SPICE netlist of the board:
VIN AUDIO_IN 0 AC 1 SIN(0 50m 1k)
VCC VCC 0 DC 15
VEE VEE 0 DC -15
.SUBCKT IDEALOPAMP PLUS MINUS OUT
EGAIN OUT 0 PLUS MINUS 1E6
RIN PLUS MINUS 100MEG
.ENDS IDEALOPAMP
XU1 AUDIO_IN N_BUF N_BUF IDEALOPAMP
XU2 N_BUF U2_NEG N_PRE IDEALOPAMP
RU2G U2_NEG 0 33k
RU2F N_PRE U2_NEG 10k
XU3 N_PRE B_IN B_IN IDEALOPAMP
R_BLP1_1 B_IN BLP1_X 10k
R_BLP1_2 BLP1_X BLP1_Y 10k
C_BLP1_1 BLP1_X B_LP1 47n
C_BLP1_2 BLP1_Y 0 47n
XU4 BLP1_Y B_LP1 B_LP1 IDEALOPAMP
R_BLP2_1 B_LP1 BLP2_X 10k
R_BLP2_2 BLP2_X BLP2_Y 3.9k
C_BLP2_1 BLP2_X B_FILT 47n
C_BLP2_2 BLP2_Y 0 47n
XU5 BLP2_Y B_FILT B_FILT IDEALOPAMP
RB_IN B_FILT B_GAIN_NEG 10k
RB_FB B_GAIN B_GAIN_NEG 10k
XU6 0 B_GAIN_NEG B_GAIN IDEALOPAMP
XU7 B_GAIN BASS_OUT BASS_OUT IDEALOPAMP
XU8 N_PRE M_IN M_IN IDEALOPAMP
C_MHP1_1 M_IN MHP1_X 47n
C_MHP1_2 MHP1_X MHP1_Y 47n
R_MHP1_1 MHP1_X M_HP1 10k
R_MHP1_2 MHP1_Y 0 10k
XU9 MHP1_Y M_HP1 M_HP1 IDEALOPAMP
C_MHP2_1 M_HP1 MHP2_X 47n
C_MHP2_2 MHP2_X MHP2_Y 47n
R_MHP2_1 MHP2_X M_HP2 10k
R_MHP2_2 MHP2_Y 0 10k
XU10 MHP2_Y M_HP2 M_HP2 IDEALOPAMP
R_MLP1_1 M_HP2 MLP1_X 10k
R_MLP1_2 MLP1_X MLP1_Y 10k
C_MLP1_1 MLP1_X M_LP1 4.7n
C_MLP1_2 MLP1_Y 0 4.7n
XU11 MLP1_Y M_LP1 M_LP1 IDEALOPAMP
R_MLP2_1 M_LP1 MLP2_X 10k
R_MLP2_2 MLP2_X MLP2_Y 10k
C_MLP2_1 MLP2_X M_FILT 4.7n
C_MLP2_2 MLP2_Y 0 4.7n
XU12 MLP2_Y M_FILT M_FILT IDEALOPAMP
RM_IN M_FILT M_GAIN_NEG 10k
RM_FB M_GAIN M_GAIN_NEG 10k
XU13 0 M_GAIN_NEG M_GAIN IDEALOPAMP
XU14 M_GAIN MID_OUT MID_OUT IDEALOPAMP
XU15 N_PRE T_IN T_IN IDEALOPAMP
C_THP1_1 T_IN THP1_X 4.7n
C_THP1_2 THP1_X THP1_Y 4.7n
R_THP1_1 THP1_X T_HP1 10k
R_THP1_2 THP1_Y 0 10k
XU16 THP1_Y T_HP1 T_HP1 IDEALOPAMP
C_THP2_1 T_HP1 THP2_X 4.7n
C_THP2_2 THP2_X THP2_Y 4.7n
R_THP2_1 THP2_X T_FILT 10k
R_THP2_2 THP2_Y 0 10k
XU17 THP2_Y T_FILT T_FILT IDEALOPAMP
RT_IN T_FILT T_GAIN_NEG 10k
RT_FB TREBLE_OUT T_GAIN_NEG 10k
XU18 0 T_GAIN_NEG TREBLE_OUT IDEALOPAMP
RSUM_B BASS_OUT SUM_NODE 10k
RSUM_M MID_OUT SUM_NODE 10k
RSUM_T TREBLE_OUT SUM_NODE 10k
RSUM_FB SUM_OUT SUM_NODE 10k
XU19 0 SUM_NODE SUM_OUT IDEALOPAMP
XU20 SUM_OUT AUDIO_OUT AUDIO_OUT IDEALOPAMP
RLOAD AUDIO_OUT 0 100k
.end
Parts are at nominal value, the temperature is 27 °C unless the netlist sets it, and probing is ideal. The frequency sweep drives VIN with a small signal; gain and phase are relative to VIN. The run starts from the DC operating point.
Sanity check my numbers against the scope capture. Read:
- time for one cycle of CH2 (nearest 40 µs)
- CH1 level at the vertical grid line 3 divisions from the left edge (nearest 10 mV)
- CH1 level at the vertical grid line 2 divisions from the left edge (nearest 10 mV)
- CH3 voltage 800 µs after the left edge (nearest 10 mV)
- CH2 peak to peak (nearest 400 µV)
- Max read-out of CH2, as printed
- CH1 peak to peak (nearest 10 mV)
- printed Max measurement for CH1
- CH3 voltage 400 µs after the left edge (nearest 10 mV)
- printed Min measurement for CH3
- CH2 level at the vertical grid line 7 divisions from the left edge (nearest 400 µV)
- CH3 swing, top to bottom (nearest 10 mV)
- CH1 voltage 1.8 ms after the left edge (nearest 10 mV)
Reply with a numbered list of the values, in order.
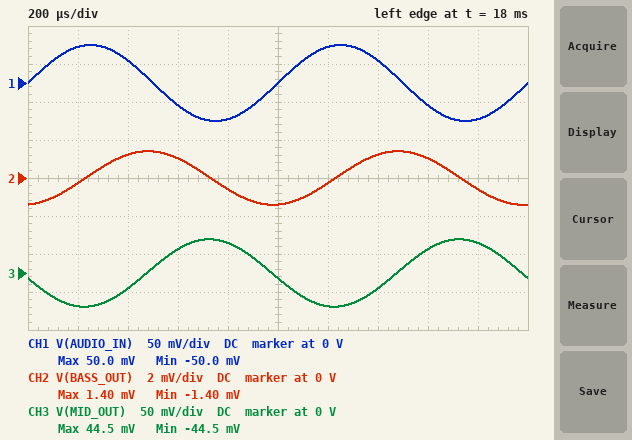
1. 1.00 ms
2. -30 mV
3. 30 mV
4. 40 mV
5. 2.8 mV
6. 1.40 mV
7. 100 mV
8. 50.0 mV
9. -20 mV
10. -44.5 mV
11. 1.2 mV
12. 90 mV
13. -50 mV
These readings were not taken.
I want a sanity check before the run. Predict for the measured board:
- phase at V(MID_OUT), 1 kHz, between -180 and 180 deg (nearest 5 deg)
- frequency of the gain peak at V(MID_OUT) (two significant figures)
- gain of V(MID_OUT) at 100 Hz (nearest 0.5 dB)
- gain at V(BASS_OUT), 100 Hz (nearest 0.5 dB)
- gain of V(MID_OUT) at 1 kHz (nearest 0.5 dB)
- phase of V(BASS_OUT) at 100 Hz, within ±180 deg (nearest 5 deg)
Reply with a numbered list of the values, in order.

1. -170 deg
2. 1.1 kHz
3. -41.5 dB
4. 1.0 dB
5. -1.0 dB
6. 125 deg
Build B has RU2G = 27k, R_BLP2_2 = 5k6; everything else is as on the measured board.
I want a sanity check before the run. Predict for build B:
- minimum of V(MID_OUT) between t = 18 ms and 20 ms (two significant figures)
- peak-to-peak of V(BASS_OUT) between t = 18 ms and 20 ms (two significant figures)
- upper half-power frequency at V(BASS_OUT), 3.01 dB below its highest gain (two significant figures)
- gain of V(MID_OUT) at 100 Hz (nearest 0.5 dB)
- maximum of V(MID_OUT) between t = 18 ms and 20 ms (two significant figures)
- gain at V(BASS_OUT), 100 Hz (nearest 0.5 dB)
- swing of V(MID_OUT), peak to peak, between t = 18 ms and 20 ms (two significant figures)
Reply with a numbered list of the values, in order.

1. -47 mV
2. 2.3 mV
3. 160 Hz
4. -41.0 dB
5. 47 mV
6. 1.5 dB
7. 93 mV
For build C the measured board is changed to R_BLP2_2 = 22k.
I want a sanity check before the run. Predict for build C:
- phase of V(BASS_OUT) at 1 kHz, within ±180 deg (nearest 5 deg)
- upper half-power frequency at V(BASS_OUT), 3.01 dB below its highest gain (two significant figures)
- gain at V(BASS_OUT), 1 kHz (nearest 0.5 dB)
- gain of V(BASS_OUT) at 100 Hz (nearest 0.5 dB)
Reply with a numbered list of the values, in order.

1. -115 deg
2. 110 Hz
3. -43.5 dB
4. -0.5 dB
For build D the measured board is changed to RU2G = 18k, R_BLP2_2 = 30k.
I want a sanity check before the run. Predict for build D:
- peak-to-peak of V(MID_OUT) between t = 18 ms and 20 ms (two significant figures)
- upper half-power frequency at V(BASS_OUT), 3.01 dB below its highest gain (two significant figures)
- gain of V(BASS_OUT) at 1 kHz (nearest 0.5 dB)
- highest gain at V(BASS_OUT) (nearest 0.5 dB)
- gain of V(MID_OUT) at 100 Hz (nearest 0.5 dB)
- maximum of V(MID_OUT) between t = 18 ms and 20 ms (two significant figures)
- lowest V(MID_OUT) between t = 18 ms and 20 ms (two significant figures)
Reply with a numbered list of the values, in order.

1. 110 mV
2. 90 Hz
3. -45.0 dB
4. 4.0 dB
5. -40.0 dB
6. 53 mV
7. -53 mV
